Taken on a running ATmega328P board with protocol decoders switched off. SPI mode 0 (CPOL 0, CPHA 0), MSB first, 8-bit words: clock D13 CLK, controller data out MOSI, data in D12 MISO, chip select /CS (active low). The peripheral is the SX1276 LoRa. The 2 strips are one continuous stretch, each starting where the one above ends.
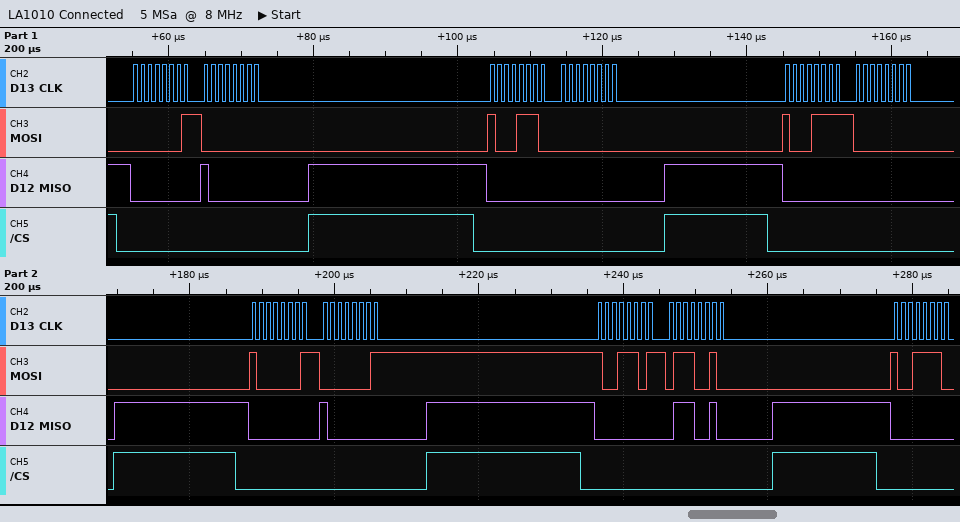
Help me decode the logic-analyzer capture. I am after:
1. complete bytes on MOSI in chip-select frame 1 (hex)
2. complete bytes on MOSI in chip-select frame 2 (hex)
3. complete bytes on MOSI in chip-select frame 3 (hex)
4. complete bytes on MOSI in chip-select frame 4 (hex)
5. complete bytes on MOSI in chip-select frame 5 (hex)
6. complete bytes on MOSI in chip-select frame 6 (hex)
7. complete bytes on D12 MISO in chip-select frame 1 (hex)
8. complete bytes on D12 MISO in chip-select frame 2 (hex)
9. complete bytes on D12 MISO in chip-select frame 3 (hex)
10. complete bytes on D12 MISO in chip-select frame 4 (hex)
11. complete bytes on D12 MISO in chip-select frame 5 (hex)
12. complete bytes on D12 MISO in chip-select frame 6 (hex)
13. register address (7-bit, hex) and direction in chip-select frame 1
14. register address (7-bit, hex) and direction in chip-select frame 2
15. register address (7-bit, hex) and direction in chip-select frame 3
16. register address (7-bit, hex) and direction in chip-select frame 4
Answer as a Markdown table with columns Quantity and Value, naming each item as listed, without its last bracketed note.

| Quantity | Value |
|---|---|
| complete bytes on MOSI in chip-select frame 1 | 01 00 |
| complete bytes on MOSI in chip-select frame 2 | 8E 00 |
| complete bytes on MOSI in chip-select frame 3 | 8F 00 |
| complete bytes on MOSI in chip-select frame 4 | 81 01 |
| complete bytes on MOSI in chip-select frame 5 | 9D 72 |
| complete bytes on MOSI in chip-select frame 6 | 9E |
| complete bytes on D12 MISO in chip-select frame 1 | 00 80 |
| complete bytes on D12 MISO in chip-select frame 2 | 00 00 |
| complete bytes on D12 MISO in chip-select frame 3 | 00 00 |
| complete bytes on D12 MISO in chip-select frame 4 | 00 80 |
| complete bytes on D12 MISO in chip-select frame 5 | 00 72 |
| complete bytes on D12 MISO in chip-select frame 6 | 00 |
| register address (7-bit, hex) and direction in chip-select frame 1 | 0x01 read |
| register address (7-bit, hex) and direction in chip-select frame 2 | 0x0E write |
| register address (7-bit, hex) and direction in chip-select frame 3 | 0x0F write |
| register address (7-bit, hex) and direction in chip-select frame 4 | 0x01 write |
